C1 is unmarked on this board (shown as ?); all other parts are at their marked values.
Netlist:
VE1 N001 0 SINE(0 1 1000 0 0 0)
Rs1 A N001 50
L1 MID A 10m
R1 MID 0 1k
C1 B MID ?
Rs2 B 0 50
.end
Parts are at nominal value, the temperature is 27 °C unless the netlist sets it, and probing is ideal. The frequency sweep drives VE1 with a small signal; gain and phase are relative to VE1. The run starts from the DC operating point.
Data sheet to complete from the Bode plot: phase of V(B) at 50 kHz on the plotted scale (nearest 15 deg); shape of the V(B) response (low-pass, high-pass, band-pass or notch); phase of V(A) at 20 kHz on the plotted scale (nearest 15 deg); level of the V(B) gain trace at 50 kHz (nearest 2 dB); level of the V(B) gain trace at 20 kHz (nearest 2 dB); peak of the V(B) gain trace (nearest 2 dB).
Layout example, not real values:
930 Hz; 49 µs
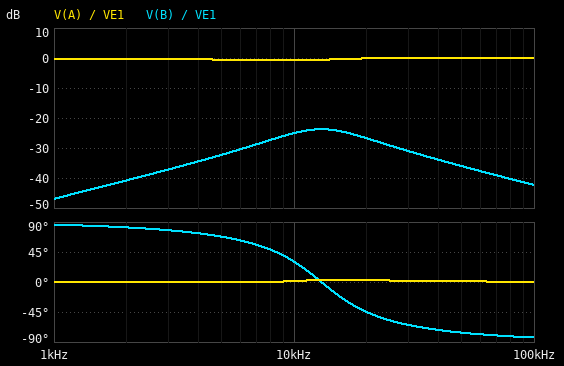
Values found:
-75 deg; band-pass; 0 deg; -36 dB; -26 dB; -24 dB
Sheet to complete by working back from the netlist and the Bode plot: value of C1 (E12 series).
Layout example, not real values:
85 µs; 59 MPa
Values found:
15 nF
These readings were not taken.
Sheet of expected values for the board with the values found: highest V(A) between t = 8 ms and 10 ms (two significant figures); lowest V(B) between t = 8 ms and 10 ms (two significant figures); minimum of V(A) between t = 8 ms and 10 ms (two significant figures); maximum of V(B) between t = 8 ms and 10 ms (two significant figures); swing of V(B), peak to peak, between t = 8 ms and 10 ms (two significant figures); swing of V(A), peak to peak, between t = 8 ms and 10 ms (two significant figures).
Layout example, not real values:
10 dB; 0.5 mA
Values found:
950 mV; -4.5 mV; -950 mV; 4.5 mV; 9.0 mV; 1.9 V
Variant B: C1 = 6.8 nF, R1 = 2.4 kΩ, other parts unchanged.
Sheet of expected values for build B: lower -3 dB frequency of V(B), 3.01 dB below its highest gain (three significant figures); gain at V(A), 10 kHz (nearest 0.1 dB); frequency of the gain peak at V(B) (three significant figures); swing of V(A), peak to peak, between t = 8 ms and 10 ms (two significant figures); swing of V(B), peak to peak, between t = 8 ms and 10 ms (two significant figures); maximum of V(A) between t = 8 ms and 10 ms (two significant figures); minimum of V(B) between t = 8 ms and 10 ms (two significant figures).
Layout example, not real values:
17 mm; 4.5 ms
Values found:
14.5 kHz; -0.3 dB; 19.3 kHz; 2.0 V; 4.2 mV; 980 mV; -2.1 mV
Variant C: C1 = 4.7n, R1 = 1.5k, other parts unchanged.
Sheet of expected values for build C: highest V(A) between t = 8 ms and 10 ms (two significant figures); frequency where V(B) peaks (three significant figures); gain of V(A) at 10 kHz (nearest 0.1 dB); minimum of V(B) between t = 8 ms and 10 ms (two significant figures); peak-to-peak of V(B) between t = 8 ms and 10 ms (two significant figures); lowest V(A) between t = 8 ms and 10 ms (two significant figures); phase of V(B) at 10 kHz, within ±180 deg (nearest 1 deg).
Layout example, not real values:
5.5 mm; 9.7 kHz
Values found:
970 mV; 23.2 kHz; -0.3 dB; -1.4 mV; 2.9 mV; -970 mV; 62 deg
